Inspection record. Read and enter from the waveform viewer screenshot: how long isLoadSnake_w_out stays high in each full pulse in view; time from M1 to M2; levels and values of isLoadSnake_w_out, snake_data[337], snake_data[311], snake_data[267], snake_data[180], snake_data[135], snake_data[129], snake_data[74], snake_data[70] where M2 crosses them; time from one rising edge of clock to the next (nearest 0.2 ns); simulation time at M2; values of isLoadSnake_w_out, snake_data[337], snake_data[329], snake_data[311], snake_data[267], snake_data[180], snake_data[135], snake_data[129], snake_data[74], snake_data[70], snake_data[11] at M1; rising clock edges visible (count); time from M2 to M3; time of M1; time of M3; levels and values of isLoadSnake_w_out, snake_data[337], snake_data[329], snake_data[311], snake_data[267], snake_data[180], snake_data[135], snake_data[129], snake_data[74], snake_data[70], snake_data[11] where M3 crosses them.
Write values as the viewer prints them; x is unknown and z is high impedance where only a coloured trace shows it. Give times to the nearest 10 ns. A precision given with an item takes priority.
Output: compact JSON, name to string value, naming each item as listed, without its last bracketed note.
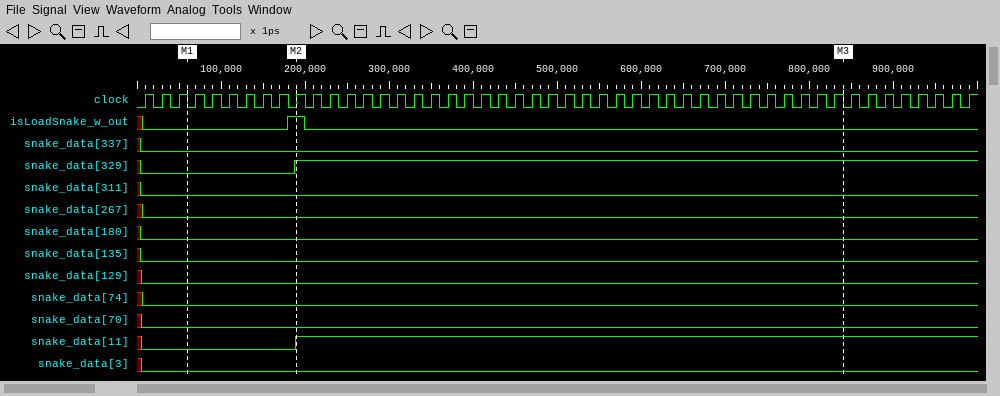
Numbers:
{"how long isLoadSnake_w_out stays high in each full pulse in view": "20 ns", "time from M1 to M2": "130 ns", "levels and values of isLoadSnake_w_out, snake_data[337], snake_data[311], snake_data[267], snake_data[180], snake_data[135], snake_data[129], snake_data[74], snake_data[70] where M2 crosses them": "isLoadSnake_w_out=1, snake_data[337]=0, snake_data[311]=0, snake_data[267]=0, snake_data[180]=0, snake_data[135]=0, snake_data[129]=0, snake_data[74]=0, snake_data[70]=0", "time from one rising edge of clock to the next": "20 ns", "simulation time at M2": "190 ns", "values of isLoadSnake_w_out, snake_data[337], snake_data[329], snake_data[311], snake_data[267], snake_data[180], snake_data[135], snake_data[129], snake_data[74], snake_data[70], snake_data[11] at M1": "isLoadSnake_w_out=0, snake_data[337]=0, snake_data[329]=0, snake_data[311]=0, snake_data[267]=0, snake_data[180]=0, snake_data[135]=0, snake_data[129]=0, snake_data[74]=0, snake_data[70]=0, snake_data[11]=0", "rising clock edges visible": "50", "time from M2 to M3": "650 ns", "time of M1": "60 ns", "time of M3": "840 ns", "levels and values of isLoadSnake_w_out, snake_data[337], snake_data[329], snake_data[311], snake_data[267], snake_data[180], snake_data[135], snake_data[129], snake_data[74], snake_data[70], snake_data[11] where M3 crosses them": "isLoadSnake_w_out=0, snake_data[337]=0, snake_data[329]=1, snake_data[311]=0, snake_data[267]=0, snake_data[180]=0, snake_data[135]=0, snake_data[129]=0, snake_data[74]=0, snake_data[70]=0, snake_data[11]=1"}
